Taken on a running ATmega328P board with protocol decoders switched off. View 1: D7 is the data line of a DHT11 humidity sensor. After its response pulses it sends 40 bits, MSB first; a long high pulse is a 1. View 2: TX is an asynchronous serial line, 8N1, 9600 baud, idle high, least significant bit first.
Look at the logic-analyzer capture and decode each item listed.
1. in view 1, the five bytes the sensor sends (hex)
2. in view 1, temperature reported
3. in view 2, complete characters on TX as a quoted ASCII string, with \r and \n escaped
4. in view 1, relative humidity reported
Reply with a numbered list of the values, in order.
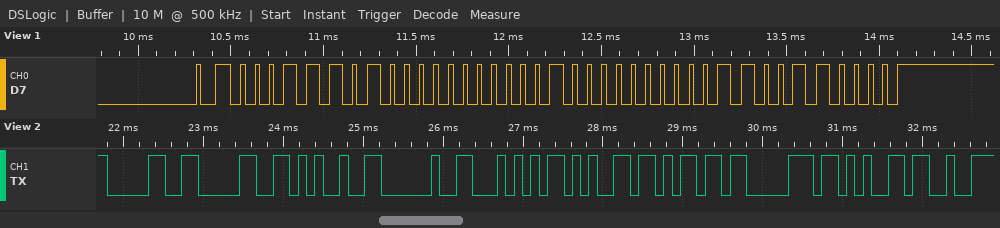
1. 1D 00 10 03 30
2. 16.3 °C
3. "00% Tempe"
4. 29 %
